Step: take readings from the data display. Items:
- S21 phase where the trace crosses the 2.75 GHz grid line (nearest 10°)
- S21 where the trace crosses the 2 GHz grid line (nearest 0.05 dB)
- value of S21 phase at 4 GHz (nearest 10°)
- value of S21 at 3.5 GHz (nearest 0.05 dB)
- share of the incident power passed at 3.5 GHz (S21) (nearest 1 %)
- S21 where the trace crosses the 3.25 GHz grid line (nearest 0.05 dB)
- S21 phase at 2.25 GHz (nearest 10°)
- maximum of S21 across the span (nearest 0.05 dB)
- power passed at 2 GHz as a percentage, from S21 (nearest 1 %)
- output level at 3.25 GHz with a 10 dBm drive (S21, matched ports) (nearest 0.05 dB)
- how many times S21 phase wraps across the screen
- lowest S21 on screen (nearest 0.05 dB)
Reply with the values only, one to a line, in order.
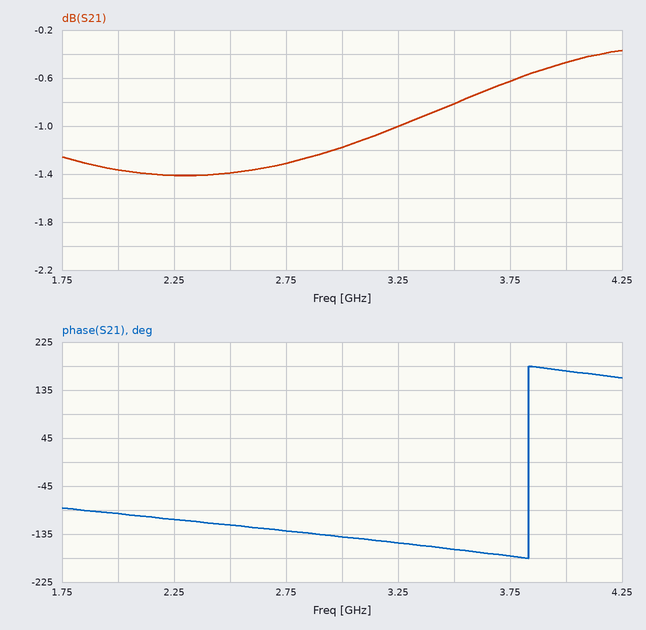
-130°
-1.35 dB
170°
-0.80 dB
83 %
-1.00 dB
-110°
-0.35 dB
73 %
9.00 dBm
1
-1.40 dB
